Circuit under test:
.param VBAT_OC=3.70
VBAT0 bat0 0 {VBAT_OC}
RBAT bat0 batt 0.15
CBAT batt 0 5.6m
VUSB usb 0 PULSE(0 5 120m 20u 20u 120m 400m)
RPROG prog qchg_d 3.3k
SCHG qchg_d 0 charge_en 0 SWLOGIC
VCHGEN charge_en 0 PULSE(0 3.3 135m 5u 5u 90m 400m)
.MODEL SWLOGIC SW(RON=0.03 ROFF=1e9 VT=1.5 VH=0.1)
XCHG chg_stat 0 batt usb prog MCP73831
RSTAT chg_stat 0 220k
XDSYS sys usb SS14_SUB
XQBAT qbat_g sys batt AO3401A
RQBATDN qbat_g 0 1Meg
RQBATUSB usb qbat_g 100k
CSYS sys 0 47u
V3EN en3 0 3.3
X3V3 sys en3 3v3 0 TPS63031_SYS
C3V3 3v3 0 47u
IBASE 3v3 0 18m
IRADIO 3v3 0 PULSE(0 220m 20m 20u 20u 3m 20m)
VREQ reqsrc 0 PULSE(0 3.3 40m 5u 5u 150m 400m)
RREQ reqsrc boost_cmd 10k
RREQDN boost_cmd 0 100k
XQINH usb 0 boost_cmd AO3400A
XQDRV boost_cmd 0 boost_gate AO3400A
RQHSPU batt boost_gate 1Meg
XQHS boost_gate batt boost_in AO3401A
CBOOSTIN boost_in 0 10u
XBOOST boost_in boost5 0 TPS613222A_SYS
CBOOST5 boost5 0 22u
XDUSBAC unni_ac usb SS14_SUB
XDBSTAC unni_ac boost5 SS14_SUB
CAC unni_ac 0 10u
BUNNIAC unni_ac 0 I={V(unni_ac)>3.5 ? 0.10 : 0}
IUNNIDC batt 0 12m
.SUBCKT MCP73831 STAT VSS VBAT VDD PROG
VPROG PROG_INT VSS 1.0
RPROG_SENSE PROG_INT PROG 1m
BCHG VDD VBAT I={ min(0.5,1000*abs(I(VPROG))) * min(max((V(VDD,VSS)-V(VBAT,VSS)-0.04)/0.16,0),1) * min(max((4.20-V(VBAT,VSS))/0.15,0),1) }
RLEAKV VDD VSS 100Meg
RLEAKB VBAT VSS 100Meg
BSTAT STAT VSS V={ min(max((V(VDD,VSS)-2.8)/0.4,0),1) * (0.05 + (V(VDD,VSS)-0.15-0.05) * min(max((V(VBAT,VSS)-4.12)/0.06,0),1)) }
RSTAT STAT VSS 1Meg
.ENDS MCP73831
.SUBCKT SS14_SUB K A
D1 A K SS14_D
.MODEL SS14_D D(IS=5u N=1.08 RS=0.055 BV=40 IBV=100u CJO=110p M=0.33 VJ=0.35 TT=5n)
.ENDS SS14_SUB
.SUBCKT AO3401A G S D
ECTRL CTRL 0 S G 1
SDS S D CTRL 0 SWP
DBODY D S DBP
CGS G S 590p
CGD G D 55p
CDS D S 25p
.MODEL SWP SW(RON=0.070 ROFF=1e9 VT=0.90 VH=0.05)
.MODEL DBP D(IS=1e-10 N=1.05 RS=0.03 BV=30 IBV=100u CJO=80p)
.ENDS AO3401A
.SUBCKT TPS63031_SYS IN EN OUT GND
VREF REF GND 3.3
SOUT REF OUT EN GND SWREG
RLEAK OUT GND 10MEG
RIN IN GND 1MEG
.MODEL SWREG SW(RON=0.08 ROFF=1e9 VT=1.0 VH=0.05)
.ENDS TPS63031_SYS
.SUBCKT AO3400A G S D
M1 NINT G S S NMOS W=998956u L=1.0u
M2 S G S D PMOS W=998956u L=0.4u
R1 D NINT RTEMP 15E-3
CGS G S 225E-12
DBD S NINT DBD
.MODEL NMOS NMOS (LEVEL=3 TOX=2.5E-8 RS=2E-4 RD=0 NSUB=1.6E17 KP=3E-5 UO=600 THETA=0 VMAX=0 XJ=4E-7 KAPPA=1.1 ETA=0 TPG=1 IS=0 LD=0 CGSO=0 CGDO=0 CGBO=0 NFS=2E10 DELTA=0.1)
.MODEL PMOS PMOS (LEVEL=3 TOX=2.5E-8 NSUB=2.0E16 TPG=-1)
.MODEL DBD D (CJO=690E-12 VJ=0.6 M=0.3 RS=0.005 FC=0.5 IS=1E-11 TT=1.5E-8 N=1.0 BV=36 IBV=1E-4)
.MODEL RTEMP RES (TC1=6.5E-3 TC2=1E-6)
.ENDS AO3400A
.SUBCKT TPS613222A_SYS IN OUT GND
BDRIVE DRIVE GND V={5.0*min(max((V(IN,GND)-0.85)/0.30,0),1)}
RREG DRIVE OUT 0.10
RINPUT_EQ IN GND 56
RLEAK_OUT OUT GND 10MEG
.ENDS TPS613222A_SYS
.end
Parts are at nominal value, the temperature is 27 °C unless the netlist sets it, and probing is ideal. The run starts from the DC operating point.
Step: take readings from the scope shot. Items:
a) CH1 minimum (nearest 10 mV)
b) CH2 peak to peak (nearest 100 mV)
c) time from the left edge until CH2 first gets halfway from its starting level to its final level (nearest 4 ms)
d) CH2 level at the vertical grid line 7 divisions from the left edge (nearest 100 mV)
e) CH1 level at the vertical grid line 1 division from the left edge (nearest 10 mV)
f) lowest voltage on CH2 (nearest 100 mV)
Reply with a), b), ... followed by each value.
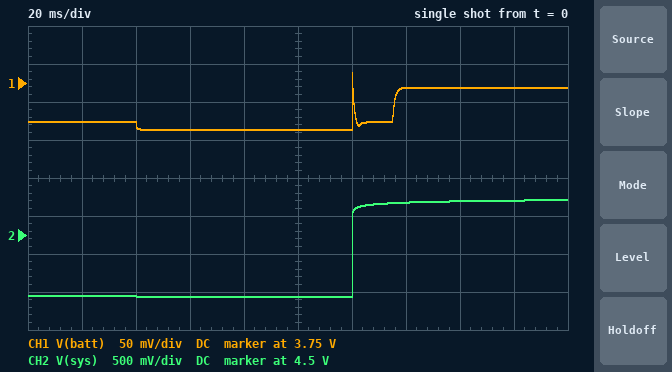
a) 3.69 V
b) 1.3 V
c) 120 ms
d) 4.9 V
e) 3.70 V
f) 3.7 V
